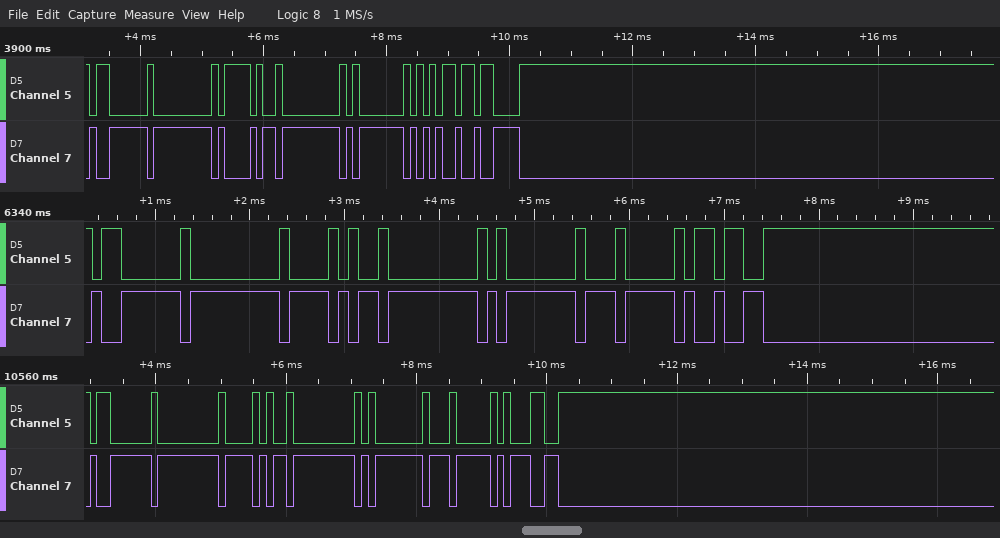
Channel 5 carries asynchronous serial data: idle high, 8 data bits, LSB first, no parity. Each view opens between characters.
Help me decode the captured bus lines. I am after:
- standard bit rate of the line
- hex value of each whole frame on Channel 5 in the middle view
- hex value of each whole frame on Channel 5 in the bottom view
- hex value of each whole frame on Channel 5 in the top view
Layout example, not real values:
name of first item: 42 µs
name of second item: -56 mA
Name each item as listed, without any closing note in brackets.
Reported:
standard bit rate of the line: 9600 baud
hex value of each whole frame on Channel 5 in the middle view: 03, 00, 28, 00, 01, 04, 9B
hex value of each whole frame on Channel 5 in the bottom view: 03, 00, 28, 00, 01, 04, 31
hex value of each whole frame on Channel 5 in the top view: 03, 00, 2F, 00, 01, B5, C3
